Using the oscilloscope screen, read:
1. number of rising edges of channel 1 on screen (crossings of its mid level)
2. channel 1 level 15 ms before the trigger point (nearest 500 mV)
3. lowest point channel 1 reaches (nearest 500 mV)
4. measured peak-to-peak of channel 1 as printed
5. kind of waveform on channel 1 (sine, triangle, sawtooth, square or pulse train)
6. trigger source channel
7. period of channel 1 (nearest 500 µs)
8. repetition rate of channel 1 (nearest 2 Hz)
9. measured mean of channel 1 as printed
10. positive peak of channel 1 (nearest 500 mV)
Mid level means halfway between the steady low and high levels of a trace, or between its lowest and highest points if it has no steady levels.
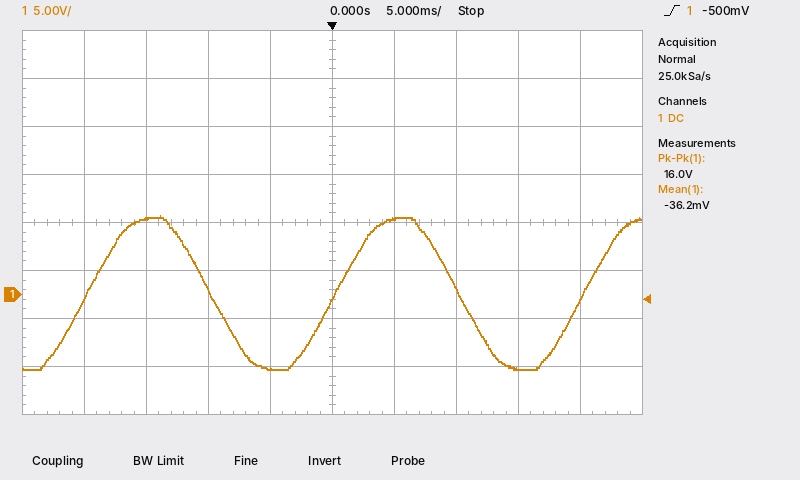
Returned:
3
8.0 V
-8.0 V
16.0 V
sine
channel 1
20.0 ms
50 Hz
-36.2 mV
8.0 V
